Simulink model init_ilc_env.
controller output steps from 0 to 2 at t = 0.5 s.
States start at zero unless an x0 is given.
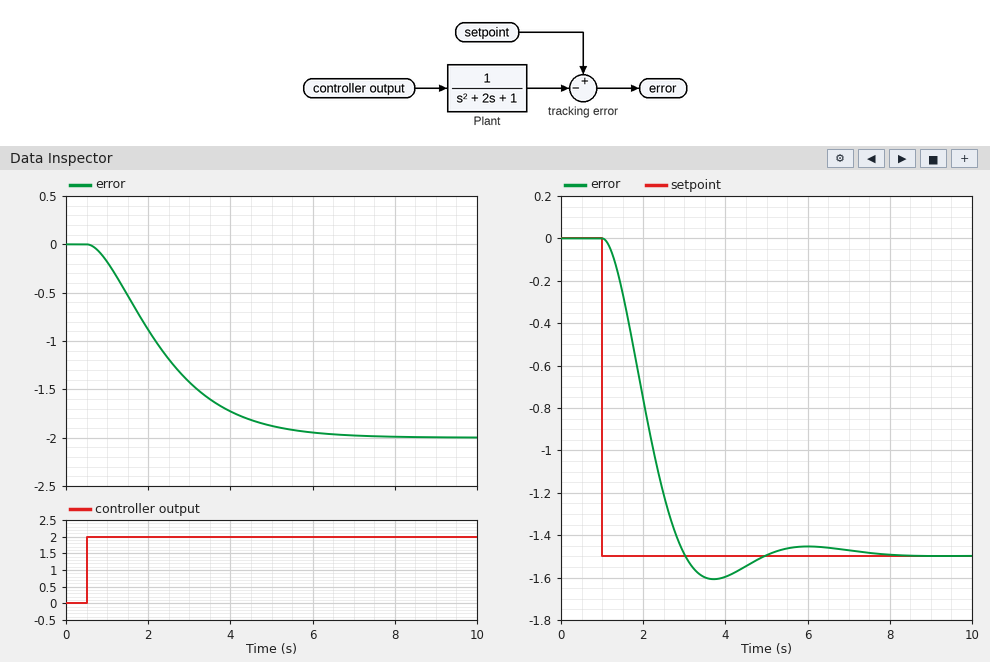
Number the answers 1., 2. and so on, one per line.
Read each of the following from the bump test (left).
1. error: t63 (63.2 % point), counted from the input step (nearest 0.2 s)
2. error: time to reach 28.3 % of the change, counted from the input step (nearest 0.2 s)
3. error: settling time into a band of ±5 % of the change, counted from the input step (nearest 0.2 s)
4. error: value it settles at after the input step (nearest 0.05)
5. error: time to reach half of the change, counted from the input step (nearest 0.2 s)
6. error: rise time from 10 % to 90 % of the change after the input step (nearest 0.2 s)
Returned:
1. 2.2 s
2. 1.0 s
3. 4.8 s
4. -2.00
5. 1.6 s
6. 3.4 s
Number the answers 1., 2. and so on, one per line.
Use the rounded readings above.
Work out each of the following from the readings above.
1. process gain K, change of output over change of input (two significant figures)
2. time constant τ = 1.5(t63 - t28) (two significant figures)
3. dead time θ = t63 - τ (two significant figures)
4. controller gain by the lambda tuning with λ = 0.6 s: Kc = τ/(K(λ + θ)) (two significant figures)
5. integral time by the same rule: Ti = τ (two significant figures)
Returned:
1. -1.0
2. 1.8 s
3. 0.40 s
4. -1.8
5. 1.8 s
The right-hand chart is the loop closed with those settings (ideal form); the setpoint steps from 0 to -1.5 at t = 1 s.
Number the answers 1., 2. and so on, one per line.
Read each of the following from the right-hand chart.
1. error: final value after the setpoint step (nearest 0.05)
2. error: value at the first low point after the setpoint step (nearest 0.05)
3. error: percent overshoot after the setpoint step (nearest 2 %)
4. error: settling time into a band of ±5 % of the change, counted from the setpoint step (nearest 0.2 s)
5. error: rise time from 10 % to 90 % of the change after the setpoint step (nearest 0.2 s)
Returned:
1. -1.50
2. -1.60
3. 8 %
4. 3.2 s
5. 1.4 s
